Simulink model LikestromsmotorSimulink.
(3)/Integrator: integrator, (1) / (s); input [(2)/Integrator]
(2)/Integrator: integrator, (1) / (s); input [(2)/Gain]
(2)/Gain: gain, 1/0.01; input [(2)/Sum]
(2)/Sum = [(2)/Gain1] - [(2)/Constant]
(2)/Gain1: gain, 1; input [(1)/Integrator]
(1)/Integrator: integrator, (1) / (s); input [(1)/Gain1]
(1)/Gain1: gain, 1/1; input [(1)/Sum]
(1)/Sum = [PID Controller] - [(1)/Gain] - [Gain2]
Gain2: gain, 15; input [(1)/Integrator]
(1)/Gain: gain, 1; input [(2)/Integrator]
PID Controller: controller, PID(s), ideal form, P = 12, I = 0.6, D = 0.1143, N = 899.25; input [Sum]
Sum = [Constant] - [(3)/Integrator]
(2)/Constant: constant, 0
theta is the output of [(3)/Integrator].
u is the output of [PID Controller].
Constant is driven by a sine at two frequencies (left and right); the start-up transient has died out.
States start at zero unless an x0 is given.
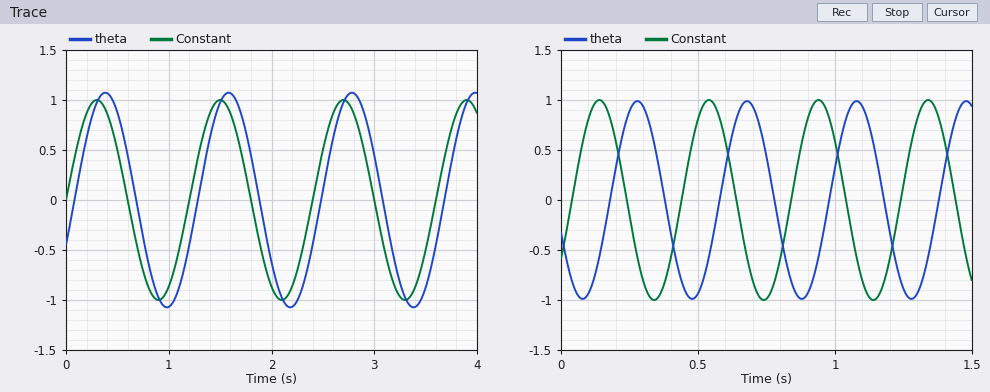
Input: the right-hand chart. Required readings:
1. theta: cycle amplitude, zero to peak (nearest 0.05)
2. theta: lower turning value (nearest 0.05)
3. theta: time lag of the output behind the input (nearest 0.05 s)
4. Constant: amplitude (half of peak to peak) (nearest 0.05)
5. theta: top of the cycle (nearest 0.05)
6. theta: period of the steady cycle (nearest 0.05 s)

1.00
-1.00
0.15 s
1.00
1.00
0.40 s
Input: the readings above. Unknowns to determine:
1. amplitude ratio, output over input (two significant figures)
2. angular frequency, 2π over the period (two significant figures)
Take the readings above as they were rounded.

1.0
16 rad/s
